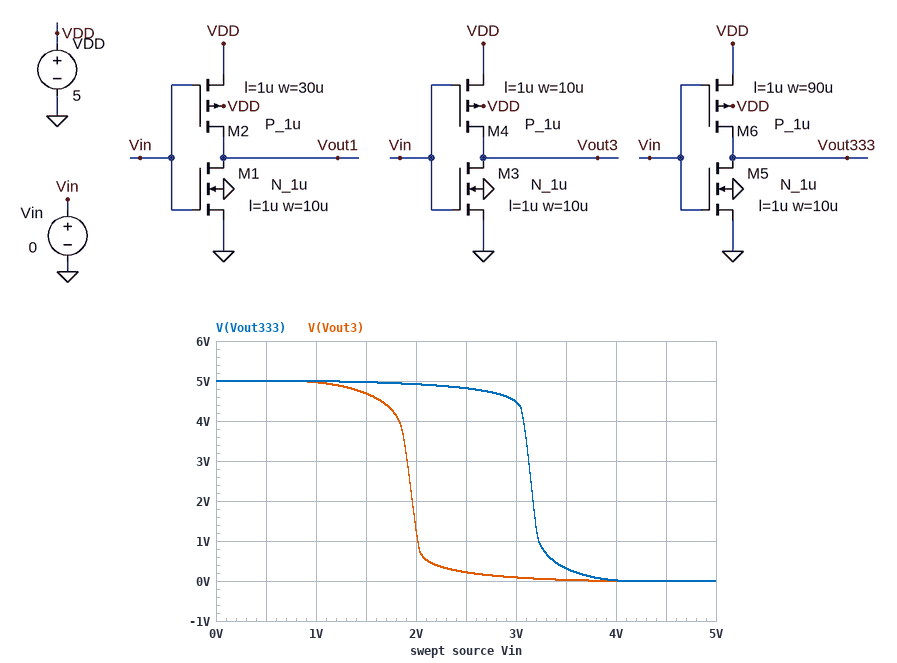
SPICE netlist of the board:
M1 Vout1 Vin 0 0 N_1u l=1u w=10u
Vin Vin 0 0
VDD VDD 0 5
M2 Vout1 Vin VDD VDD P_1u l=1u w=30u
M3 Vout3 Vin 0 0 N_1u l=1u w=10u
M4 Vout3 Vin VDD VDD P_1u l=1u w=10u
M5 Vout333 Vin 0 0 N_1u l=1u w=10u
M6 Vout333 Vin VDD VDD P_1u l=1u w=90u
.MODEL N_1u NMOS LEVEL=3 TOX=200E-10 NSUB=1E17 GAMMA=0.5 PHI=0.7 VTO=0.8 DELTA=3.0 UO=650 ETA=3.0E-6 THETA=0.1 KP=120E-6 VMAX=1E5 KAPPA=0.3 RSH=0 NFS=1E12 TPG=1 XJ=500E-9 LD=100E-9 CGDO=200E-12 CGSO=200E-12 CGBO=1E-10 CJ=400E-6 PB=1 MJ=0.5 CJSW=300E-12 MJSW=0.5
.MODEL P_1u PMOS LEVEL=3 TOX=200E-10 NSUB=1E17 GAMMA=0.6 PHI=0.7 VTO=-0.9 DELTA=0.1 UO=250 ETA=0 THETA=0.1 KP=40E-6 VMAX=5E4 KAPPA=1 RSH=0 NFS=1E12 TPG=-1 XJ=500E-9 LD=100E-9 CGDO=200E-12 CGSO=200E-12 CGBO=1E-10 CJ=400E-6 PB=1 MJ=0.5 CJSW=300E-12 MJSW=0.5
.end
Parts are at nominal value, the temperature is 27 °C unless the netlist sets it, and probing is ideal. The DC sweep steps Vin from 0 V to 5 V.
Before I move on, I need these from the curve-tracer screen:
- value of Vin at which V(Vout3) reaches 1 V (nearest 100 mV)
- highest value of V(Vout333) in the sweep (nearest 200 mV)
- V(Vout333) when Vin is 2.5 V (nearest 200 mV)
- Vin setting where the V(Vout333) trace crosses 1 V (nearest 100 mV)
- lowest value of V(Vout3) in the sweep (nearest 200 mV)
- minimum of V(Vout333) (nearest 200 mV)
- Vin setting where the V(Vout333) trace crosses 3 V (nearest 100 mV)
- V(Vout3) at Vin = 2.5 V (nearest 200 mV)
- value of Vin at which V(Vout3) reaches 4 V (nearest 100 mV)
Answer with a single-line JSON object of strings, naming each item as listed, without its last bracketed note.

{"value of Vin at which V(Vout3) reaches 1 V": "2.0 V", "highest value of V(Vout333) in the sweep": "5.0 V", "V(Vout333) when Vin is 2.5 V": "4.8 V", "Vin setting where the V(Vout333) trace crosses 1 V": "3.2 V", "lowest value of V(Vout3) in the sweep": "0 V", "minimum of V(Vout333)": "0 V", "Vin setting where the V(Vout333) trace crosses 3 V": "3.1 V", "V(Vout3) at Vin = 2.5 V": "200 mV", "value of Vin at which V(Vout3) reaches 4 V": "1.8 V"}
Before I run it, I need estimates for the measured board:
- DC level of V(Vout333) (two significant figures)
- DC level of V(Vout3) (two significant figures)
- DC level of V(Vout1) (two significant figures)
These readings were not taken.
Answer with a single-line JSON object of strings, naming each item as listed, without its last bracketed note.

{"DC level of V(Vout333)": "5.0 V", "DC level of V(Vout3)": "5.0 V", "DC level of V(Vout1)": "5.0 V"}
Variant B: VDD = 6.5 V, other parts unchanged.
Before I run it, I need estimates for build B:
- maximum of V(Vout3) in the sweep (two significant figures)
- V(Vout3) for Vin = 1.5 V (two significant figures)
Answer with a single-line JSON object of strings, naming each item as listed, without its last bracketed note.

{"maximum of V(Vout3) in the sweep": "6.5 V", "V(Vout3) for Vin = 1.5 V": "6.3 V"}
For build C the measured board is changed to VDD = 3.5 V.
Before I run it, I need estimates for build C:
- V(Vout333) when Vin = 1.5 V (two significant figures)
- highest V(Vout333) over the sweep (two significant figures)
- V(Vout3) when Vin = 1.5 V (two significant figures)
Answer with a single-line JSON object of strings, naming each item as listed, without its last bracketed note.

{"V(Vout333) when Vin = 1.5 V": "3.4 V", "highest V(Vout333) over the sweep": "3.5 V", "V(Vout3) when Vin = 1.5 V": "360 mV"}
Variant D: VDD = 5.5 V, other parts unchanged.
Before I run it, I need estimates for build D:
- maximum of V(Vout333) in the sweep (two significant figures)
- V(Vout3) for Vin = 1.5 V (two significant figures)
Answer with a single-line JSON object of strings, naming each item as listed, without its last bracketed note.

{"maximum of V(Vout333) in the sweep": "5.5 V", "V(Vout3) for Vin = 1.5 V": "5.2 V"}
